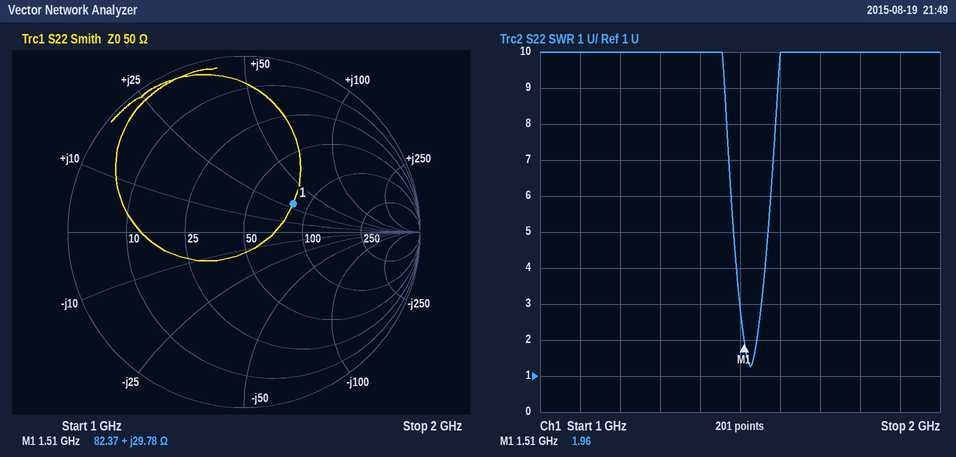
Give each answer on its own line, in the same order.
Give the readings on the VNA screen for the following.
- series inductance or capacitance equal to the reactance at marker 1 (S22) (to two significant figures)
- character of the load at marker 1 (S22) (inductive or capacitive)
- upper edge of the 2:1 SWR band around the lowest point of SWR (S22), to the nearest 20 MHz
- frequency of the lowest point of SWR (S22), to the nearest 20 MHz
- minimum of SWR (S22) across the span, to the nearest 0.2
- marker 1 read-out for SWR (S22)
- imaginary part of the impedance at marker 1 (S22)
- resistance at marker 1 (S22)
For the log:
3.1 nH
inductive
1.54 GHz
1.52 GHz
1.2
1.96
+29.78 Ω
82.37 Ω
